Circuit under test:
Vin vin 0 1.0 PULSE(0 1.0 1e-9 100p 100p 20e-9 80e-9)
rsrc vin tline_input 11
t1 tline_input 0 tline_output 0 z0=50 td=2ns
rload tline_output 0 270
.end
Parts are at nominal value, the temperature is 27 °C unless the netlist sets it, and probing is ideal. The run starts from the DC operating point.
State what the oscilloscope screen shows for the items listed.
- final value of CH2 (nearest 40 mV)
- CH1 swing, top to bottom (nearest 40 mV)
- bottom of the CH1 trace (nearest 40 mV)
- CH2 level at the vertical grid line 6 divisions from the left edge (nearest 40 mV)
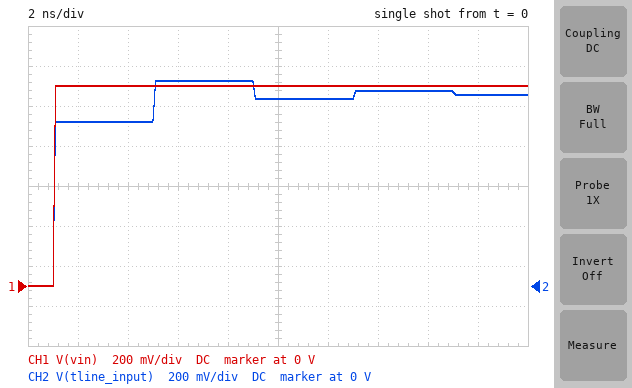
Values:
960 mV
1.00 V
0 V
920 mV
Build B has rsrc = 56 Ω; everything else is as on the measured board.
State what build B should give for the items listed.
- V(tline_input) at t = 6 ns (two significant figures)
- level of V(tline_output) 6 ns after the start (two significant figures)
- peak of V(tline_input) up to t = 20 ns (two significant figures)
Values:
810 mV
800 mV
830 mV
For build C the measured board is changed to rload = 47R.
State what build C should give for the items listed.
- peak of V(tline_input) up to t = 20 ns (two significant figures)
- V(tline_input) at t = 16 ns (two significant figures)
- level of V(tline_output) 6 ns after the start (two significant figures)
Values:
820 mV
810 mV
790 mV
